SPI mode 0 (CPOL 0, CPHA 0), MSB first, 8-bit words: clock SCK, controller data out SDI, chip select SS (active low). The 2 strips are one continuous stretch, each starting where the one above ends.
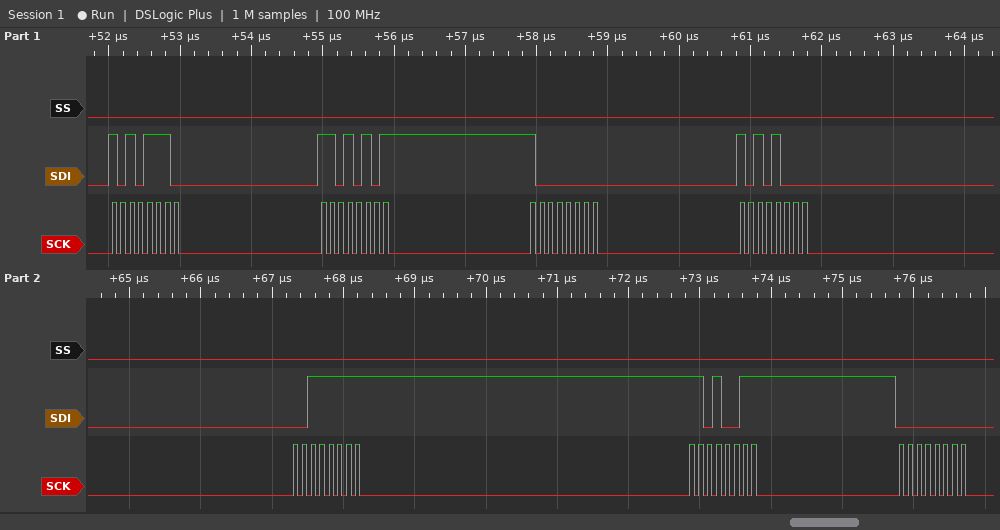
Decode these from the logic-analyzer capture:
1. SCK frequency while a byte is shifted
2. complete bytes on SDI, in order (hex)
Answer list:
8 MHz
AE D5 80 A8 3F D3 00
